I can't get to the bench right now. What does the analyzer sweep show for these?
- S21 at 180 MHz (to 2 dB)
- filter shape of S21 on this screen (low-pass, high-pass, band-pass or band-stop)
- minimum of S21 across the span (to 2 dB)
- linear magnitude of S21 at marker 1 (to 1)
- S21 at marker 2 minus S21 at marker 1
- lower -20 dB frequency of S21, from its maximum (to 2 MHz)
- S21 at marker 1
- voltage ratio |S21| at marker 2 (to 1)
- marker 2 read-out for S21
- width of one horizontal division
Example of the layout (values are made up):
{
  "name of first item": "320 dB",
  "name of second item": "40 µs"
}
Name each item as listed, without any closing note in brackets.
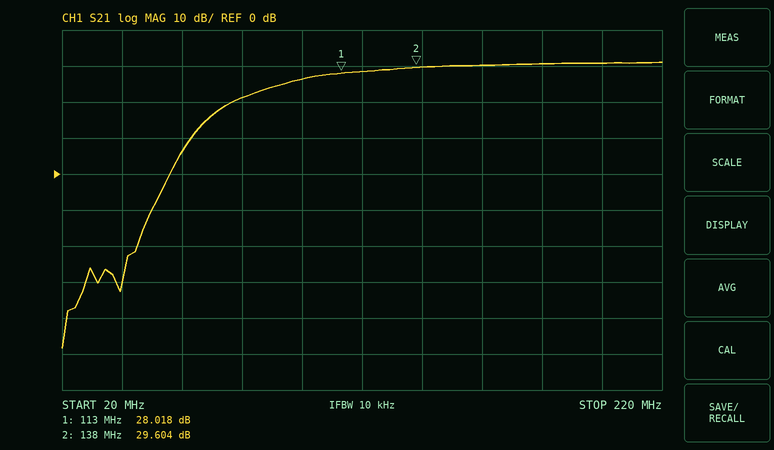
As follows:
{
  "S21 at 180 MHz": "30 dB",
  "filter shape of S21 on this screen": "high-pass",
  "minimum of S21 across the span": "-48 dB",
  "linear magnitude of S21 at marker 1": "25",
  "S21 at marker 2 minus S21 at marker 1": "1.586 dB",
  "lower -20 dB frequency of S21, from its maximum": "64 MHz",
  "S21 at marker 1": "28.018 dB",
  "voltage ratio |S21| at marker 2": "30",
  "marker 2 read-out for S21": "29.604 dB",
  "width of one horizontal division": "20 MHz"
}
